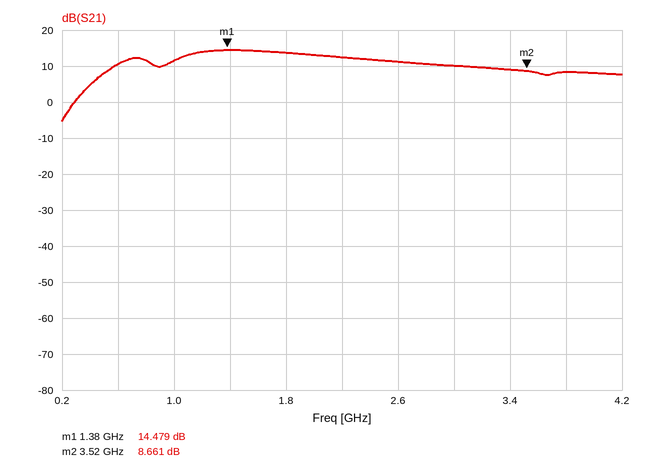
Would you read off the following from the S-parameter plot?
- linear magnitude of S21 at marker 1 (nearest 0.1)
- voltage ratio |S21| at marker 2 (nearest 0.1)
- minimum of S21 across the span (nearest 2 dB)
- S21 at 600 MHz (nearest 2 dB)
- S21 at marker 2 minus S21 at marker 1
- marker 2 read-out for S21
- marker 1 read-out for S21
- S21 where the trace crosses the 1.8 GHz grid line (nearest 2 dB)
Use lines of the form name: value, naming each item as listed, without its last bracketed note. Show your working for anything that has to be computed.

linear magnitude of S21 at marker 1: 10^(14.479/20) ≈ 5.3
voltage ratio |S21| at marker 2: 10^(8.661/20) ≈ 2.7
minimum of S21 across the span: -6 dB
S21 at 600 MHz: 10 dB
S21 at marker 2 minus S21 at marker 1: 8.661 − (14.479) = -5.818 dB
marker 2 read-out for S21: 8.661 dB
marker 1 read-out for S21: 14.479 dB
S21 where the trace crosses the 1.8 GHz grid line: 14 dB
